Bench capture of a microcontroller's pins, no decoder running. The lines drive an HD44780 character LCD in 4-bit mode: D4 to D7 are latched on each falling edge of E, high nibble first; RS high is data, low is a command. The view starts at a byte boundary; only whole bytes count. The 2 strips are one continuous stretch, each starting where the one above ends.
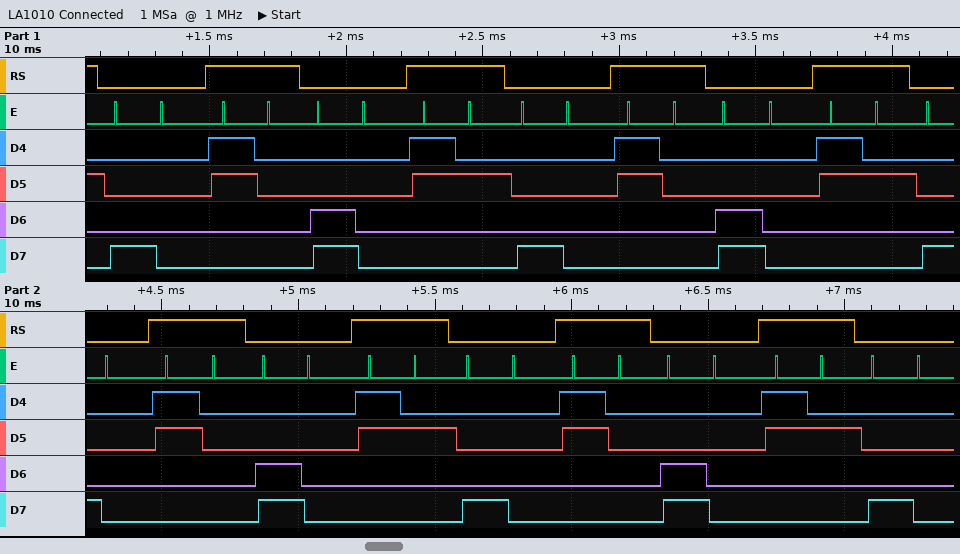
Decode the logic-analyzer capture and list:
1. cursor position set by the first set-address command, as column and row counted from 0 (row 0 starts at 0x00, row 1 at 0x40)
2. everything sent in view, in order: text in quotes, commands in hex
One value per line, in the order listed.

column 0, row 0
0x80 "0" 0xC0 "2" 0x80 "0" 0xC0 "2" 0x80 "0" 0xC0 "2" 0x80 "0" 0xC0 "2" 0x80
